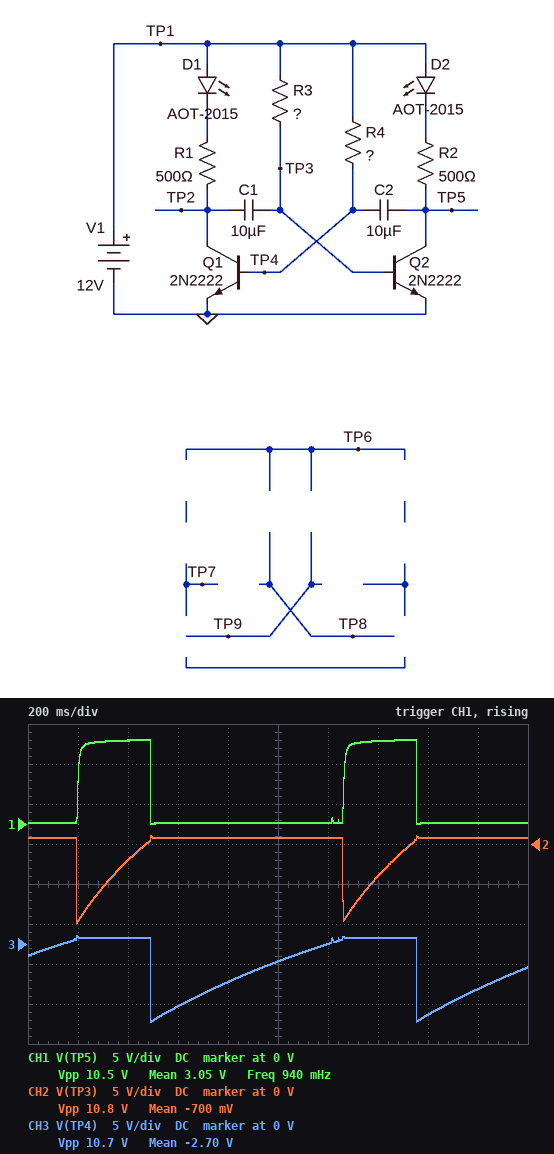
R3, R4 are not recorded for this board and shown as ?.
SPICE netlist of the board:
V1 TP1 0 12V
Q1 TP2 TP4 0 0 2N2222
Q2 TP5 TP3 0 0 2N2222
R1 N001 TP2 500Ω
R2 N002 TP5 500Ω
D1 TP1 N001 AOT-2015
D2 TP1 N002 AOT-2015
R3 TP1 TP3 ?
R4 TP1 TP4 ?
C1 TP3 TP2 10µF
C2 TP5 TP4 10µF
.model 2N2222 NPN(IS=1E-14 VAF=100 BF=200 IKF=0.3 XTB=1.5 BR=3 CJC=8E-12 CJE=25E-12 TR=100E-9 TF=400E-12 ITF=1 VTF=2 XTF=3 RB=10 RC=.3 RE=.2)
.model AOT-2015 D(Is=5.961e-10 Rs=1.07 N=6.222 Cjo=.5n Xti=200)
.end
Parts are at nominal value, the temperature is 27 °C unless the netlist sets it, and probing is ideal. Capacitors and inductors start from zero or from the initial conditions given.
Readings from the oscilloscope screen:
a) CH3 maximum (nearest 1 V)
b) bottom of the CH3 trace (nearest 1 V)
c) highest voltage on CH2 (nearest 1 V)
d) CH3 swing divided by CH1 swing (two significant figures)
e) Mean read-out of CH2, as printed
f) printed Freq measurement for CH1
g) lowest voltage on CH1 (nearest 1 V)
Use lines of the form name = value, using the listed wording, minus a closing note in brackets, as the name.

CH3 maximum = 1 V
bottom of the CH3 trace = -10 V
highest voltage on CH2 = 1 V
CH3 swing divided by CH1 swing = 1.0
Mean read-out of CH2, as printed = -700 mV
printed Freq measurement for CH1 = 940 mHz
lowest voltage on CH1 = 0 V
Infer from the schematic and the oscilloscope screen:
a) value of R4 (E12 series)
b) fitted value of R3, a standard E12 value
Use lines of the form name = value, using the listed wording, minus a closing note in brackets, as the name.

value of R4 = 120 kΩ
fitted value of R3, a standard E12 value = 47 kΩ
